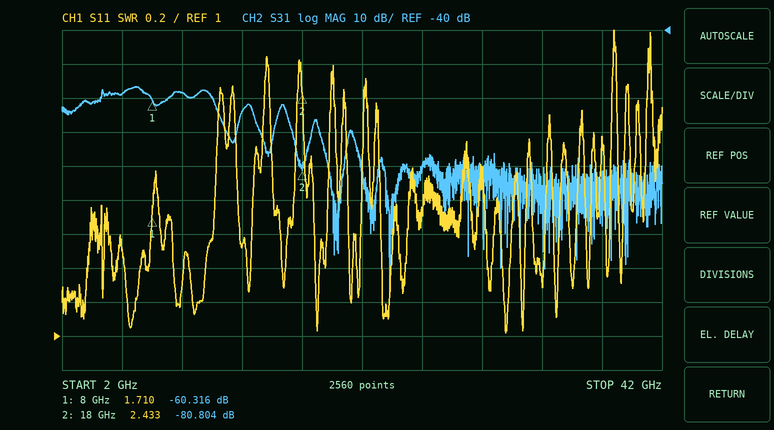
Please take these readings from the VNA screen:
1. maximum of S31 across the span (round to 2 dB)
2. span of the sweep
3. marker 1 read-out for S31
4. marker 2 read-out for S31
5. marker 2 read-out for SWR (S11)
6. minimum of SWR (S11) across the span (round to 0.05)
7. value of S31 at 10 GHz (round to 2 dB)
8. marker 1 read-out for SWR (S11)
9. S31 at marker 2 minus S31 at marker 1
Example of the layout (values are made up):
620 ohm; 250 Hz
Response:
-56 dB; 40 GHz; -60.316 dB; -80.804 dB; 2.433; 1.00; -58 dB; 1.710; -20.488 dB
